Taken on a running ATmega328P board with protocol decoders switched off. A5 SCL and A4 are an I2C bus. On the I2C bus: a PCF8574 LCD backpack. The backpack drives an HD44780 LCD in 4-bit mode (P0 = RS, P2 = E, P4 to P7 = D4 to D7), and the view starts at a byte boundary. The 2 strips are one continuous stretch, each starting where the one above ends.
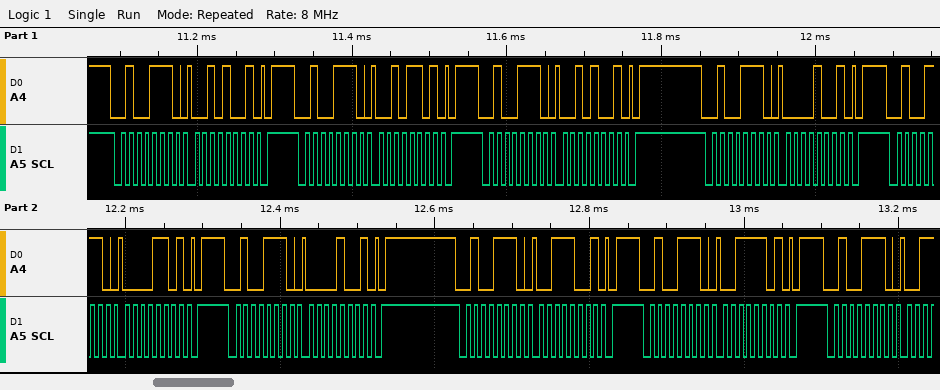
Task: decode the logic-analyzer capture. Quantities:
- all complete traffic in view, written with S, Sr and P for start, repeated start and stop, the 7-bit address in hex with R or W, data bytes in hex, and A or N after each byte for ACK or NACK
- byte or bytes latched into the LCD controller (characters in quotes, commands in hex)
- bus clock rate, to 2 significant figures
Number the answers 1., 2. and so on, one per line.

1. S 27W A 29 A P S 27W A 2D A P S 27W A 29 A P S 27W A 09 A P S 27W A 0D A P S 27W A 09 A P S 27W A 39 A P S 27W A 3D A P S 27W A
2. ' '
3. 100 kHz
